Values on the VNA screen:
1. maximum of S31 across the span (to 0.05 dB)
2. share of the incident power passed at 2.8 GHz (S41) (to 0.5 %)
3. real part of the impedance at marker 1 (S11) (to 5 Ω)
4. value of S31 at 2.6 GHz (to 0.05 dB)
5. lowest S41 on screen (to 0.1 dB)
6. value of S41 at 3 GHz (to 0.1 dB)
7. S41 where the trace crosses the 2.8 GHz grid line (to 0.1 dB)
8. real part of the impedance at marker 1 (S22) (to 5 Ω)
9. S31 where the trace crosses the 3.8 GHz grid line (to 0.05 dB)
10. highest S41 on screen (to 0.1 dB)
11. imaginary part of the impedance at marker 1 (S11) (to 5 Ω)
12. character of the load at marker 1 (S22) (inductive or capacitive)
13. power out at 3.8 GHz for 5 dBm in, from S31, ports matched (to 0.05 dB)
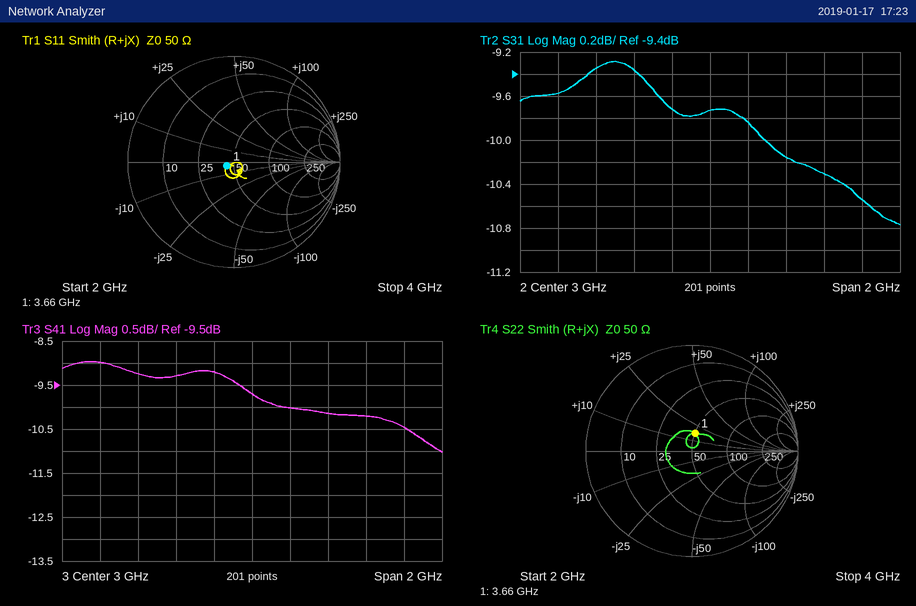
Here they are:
-9.30 dB
12.0 %
45 Ω
-9.35 dB
-11.0 dB
-9.7 dB
-9.2 dB
50 Ω
-10.55 dB
-9.0 dB
-5 Ω
inductive
-5.55 dBm
